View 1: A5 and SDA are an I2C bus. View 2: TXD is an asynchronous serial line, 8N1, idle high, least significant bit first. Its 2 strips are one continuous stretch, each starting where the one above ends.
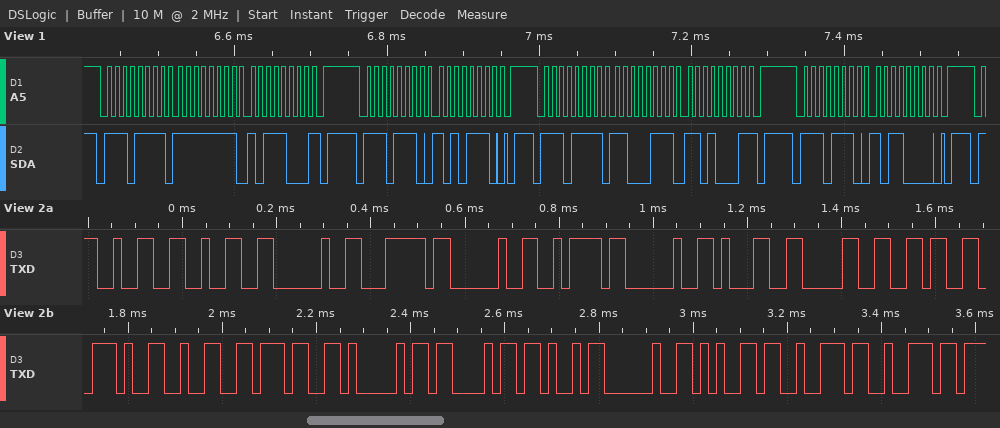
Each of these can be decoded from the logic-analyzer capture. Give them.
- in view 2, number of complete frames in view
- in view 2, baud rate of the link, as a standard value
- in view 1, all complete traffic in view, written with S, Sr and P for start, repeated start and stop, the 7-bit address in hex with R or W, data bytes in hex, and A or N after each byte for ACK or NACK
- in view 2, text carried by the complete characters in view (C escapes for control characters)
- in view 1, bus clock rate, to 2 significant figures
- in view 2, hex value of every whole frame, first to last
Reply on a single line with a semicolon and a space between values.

20; 57600 baud; S 77R A FF A B8 N P S 77W A AE A P S 77R A C7 A D1 N P S 77W A B0 A P; "22 | z 106.27ACK err"; 100 kHz; 32 32 20 7C 20 7A 20 31 30 36 2E 32 37 41 43 4B 20 65 72 72
